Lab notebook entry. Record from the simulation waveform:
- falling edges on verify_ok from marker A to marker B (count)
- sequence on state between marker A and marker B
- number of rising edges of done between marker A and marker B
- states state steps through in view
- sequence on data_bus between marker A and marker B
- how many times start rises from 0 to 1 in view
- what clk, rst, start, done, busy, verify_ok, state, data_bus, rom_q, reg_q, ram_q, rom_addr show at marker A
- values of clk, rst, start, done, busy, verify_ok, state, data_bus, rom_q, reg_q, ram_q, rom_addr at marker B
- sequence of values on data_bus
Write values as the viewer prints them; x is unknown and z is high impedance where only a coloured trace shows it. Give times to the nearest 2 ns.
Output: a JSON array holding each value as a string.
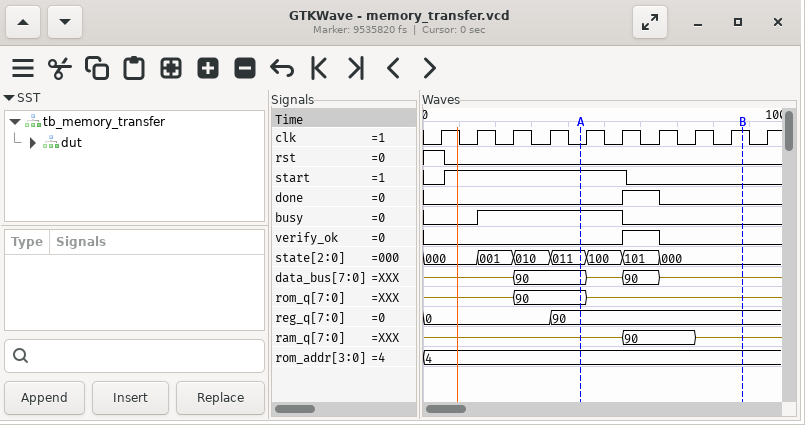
["1", "011, 100, 101, 000", "1", "000, 001, 010, 011, 100, 101, 000", "90, z, 90, z", "1", "clk=0, rst=0, start=1, done=0, busy=1, verify_ok=0, state=011, data_bus=90, rom_q=90, reg_q=90, ram_q=z, rom_addr=4", "clk=1, rst=0, start=0, done=0, busy=0, verify_ok=0, state=000, data_bus=z, rom_q=z, reg_q=90, ram_q=z, rom_addr=4", "z, 90, z, 90, z"]
